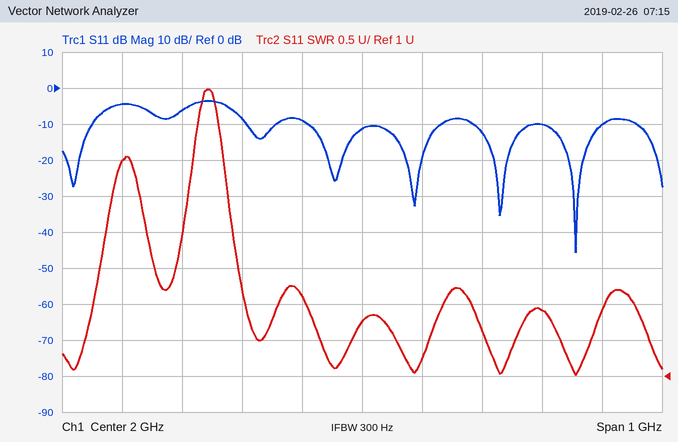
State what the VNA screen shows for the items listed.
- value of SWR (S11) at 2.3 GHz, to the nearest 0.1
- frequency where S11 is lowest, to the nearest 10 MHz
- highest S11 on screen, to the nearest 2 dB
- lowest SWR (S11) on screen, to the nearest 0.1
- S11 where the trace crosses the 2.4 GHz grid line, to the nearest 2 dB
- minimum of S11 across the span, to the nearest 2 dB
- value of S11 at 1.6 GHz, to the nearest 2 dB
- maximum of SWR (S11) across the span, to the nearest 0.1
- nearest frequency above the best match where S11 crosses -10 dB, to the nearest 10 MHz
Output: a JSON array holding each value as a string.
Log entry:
["1.9", "2.36 GHz", "-4 dB", "1.0", "-10 dB", "-46 dB", "-4 dB", "5.0", "2.40 GHz"]
